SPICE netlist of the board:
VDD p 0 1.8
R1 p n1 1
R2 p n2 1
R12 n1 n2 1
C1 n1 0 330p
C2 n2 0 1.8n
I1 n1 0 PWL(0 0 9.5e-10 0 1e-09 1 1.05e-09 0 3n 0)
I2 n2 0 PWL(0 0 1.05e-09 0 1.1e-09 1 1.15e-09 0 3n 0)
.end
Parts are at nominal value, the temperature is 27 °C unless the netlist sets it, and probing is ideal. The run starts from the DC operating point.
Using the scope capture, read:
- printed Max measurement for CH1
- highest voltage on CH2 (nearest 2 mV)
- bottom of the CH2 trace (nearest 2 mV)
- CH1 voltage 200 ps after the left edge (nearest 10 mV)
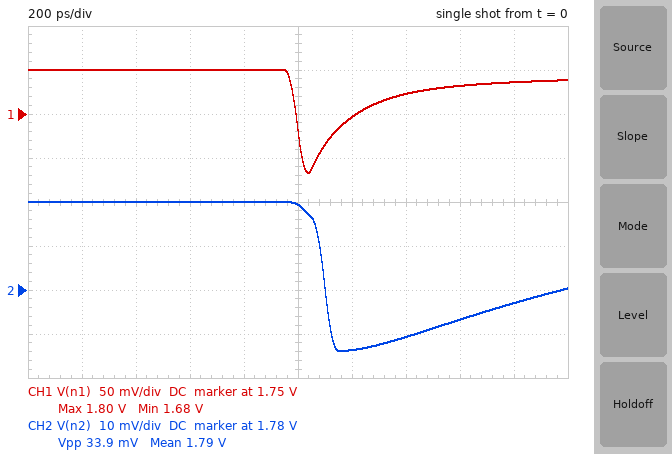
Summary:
1.80 V
1.800 V
1.766 V
1.80 V
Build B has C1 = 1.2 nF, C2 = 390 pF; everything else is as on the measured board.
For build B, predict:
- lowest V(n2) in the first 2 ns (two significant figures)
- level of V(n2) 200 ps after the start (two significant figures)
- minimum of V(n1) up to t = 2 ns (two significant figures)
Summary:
1.7 V
1.8 V
1.8 V
